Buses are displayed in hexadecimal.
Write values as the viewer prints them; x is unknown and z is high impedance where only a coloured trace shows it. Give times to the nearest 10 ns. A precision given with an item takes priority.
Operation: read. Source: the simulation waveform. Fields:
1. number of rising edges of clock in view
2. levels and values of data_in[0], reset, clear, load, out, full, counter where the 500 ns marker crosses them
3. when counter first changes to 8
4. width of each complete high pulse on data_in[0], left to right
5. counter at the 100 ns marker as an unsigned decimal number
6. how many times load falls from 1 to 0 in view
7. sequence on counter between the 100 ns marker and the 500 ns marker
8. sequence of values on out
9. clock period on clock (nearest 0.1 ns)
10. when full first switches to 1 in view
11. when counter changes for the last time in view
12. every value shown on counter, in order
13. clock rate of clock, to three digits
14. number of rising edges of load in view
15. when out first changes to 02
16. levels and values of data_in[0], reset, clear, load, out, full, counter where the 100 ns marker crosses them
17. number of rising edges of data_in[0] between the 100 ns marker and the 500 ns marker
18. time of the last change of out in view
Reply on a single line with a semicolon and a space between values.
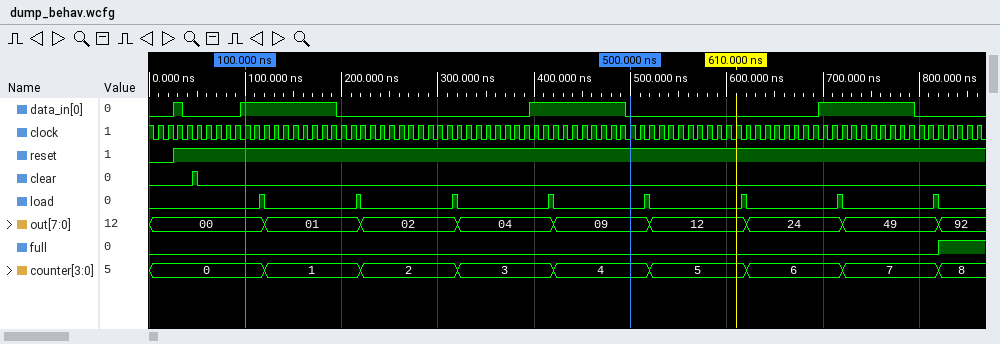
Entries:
86; data_in[0]=0, reset=1, clear=0, load=0, out=09, full=0, counter=4; 820 ns; 10 ns, 100 ns, 100 ns, 100 ns; 0; 8; 0, 1, 2, 3, 4; 00, 01, 02, 04, 09, 12, 24, 49, 92; 10 ns; 820 ns; 820 ns; 0, 1, 2, 3, 4, 5, 6, 7, 8; 100 MHz; 8; 220 ns; data_in[0]=1, reset=1, clear=0, load=0, out=00, full=0, counter=0; 1; 820 ns
